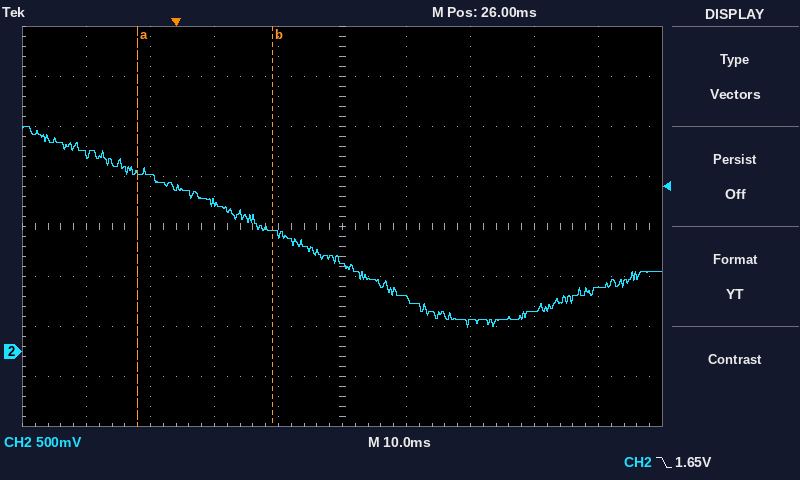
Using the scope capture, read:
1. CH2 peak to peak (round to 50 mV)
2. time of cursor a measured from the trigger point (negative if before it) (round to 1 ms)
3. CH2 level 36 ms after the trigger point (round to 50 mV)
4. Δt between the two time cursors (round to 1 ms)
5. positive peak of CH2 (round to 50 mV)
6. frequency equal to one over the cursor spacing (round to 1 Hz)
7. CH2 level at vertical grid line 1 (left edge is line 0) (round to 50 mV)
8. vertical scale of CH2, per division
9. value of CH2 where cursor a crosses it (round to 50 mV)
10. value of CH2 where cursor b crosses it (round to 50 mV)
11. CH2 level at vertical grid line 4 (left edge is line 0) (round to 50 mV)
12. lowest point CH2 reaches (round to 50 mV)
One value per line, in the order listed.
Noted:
2.00 V
-6 ms
550 mV
21 ms
2.25 V
48 Hz
1.95 V
500 mV
1.80 V
1.20 V
1.15 V
250 mV
